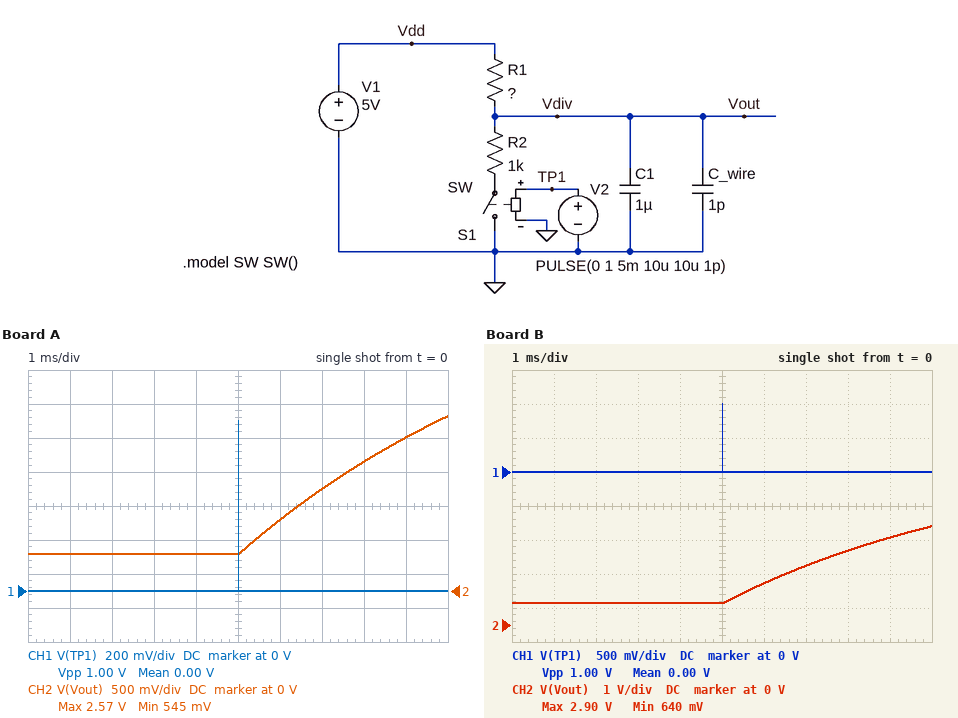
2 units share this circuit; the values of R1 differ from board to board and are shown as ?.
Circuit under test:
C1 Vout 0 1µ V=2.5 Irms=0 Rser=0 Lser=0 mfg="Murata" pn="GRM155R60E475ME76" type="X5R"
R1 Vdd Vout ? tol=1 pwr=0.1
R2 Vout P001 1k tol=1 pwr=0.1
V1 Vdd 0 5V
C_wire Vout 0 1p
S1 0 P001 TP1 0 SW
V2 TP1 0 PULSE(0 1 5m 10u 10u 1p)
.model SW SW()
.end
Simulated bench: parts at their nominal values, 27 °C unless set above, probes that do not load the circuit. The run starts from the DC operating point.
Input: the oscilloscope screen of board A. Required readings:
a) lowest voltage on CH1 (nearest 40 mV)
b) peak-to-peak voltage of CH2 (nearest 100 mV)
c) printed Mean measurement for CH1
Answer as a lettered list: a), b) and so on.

a) 0 V
b) 2.0 V
c) 0.00 V
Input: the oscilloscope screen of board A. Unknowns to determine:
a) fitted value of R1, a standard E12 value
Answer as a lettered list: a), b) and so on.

a) 8.2 kΩ
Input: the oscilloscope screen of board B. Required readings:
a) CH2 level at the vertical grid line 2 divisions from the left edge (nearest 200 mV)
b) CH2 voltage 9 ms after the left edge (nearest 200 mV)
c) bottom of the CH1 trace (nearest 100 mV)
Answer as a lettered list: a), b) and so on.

a) 600 mV
b) 2.6 V
c) 0 V
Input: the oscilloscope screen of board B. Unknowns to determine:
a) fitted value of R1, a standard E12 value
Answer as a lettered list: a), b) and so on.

a) 6.8 kΩ
